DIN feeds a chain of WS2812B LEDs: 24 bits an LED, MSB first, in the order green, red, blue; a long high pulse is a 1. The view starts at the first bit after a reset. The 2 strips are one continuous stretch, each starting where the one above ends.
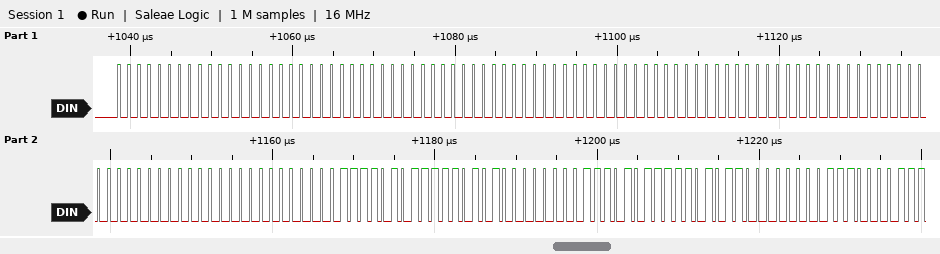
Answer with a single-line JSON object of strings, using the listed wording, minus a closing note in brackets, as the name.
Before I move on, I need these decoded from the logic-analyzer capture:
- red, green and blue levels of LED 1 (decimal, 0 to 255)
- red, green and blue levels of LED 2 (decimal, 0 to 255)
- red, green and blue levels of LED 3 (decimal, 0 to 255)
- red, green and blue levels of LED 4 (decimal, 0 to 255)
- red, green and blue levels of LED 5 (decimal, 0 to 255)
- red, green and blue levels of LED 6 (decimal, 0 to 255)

{"red, green and blue levels of LED 1": "0, 0, 0", "red, green and blue levels of LED 2": "0, 0, 0", "red, green and blue levels of LED 3": "0, 0, 0", "red, green and blue levels of LED 4": "0, 0, 0", "red, green and blue levels of LED 5": "245, 0, 245", "red, green and blue levels of LED 6": "235, 0, 235"}
